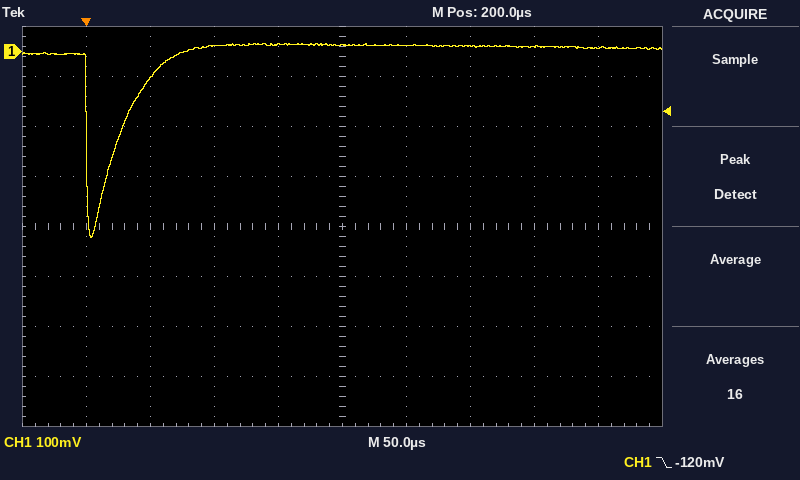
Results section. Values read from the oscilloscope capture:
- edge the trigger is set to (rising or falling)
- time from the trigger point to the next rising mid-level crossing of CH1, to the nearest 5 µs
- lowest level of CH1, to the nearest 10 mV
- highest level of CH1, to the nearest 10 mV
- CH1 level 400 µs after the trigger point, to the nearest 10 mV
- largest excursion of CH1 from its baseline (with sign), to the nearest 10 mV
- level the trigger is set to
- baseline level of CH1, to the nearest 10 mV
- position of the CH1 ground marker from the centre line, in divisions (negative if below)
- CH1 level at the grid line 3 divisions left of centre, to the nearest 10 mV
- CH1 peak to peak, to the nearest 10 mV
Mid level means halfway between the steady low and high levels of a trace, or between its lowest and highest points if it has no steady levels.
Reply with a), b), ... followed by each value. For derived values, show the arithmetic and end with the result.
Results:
a) falling
b) 25 µs
c) -370 mV
d) 20 mV
e) 10 mV
f) -370 mV − (10 mV) = -380 mV
g) -120 mV
h) 10 mV
i) +3.5 div
j) -50 mV
k) 20 mV − (-370 mV) = 390 mV
